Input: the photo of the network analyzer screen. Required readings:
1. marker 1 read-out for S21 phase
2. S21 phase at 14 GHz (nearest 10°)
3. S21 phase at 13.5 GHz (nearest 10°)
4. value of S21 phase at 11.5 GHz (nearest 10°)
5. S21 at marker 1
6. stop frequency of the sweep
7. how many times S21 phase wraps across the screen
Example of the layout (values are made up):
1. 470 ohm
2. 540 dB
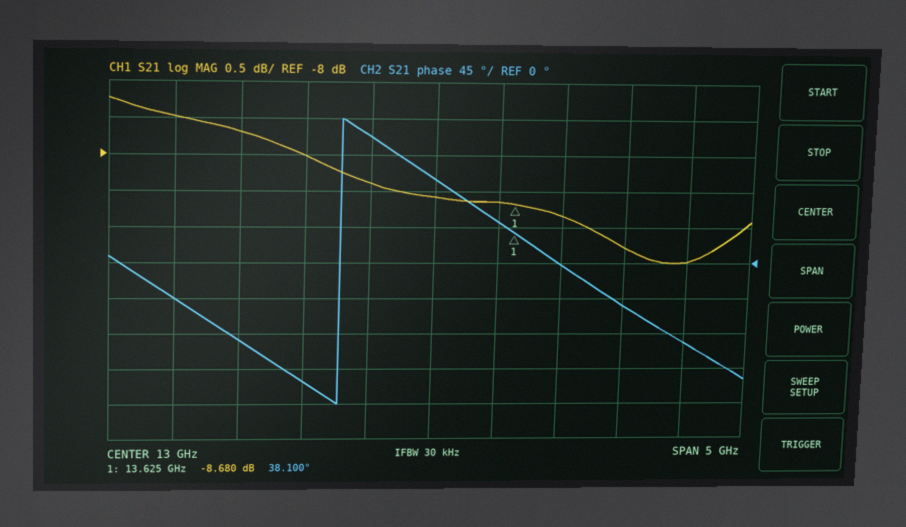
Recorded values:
1. 38.100°
2. 0°
3. 50°
4. -100°
5. -8.680 dB
6. 15.5 GHz
7. 1
